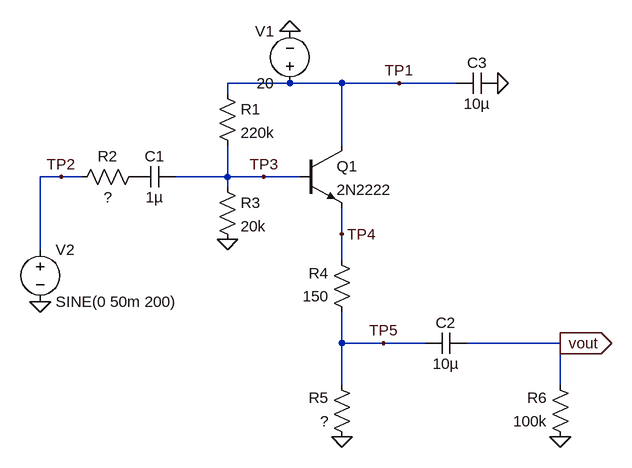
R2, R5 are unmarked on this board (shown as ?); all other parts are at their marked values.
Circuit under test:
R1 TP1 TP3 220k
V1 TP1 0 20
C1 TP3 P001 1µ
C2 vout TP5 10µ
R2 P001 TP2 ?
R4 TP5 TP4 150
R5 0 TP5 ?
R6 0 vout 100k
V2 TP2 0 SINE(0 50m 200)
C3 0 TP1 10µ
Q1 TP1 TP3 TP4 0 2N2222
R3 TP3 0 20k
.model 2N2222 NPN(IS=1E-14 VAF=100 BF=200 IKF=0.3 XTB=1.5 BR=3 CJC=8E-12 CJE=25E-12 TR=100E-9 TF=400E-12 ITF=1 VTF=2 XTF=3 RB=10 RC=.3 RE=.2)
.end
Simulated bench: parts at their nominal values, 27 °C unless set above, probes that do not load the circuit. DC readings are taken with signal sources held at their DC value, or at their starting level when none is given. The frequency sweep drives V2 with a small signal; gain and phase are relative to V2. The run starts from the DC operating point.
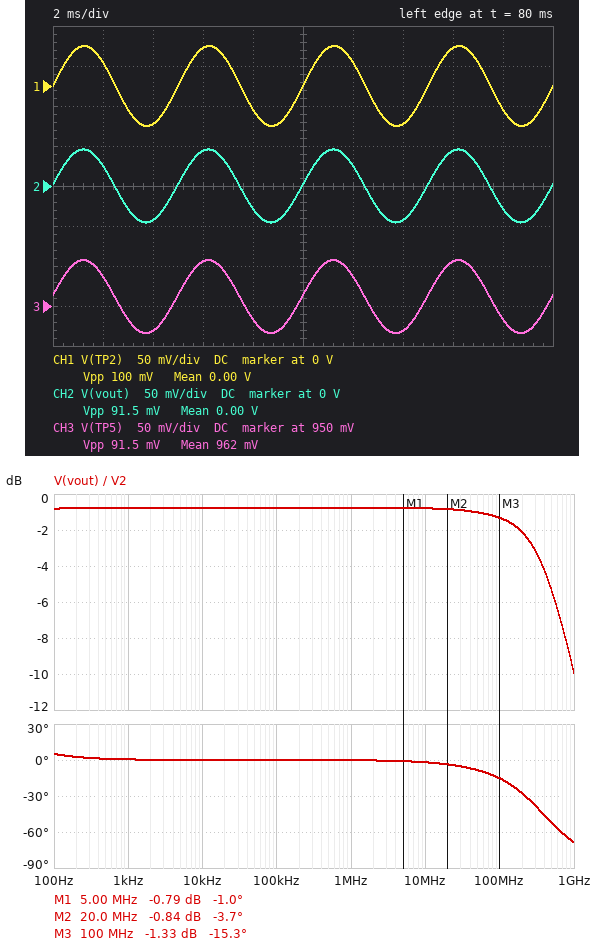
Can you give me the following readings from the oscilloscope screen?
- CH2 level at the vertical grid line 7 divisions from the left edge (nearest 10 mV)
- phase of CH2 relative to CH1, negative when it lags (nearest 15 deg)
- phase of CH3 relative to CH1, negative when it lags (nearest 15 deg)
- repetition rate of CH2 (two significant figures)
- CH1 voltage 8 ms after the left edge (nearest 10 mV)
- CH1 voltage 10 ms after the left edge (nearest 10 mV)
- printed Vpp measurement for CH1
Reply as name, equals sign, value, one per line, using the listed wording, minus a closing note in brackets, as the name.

CH2 level at the vertical grid line 7 divisions from the left edge = -40 mV
phase of CH2 relative to CH1, negative when it lags = 0 deg
phase of CH3 relative to CH1, negative when it lags = 0 deg
repetition rate of CH2 = 200 Hz
CH1 voltage 8 ms after the left edge = -30 mV
CH1 voltage 10 ms after the left edge = 0 V
printed Vpp measurement for CH1 = 100 mV
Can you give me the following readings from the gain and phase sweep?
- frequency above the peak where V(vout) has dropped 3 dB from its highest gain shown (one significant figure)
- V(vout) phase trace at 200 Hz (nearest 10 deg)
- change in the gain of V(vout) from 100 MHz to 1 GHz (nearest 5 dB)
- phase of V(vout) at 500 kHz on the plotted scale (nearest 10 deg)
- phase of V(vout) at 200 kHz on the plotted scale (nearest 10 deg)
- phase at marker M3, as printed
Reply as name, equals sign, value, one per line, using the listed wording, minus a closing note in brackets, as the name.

frequency above the peak where V(vout) has dropped 3 dB from its highest gain shown = 400 MHz
V(vout) phase trace at 200 Hz = 0 deg
change in the gain of V(vout) from 100 MHz to 1 GHz = -10 dB
phase of V(vout) at 500 kHz on the plotted scale = 0 deg
phase of V(vout) at 200 kHz on the plotted scale = 0 deg
phase at marker M3, as printed = -15.3 deg
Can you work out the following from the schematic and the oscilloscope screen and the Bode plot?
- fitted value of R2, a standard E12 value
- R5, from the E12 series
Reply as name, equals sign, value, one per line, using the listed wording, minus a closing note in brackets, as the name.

fitted value of R2, a standard E12 value = 150 Ω
R5, from the E12 series = 2.7 kΩ
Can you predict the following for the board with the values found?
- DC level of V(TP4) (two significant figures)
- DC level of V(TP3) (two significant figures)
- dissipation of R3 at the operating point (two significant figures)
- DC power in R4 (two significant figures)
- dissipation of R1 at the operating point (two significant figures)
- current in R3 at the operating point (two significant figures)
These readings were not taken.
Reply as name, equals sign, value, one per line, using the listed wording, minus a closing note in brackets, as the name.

DC level of V(TP4) = 1.0 V
DC level of V(TP3) = 1.6 V
dissipation of R3 at the operating point = 130 µW
DC power in R4 = 19 µW
dissipation of R1 at the operating point = 1.5 mW
current in R3 at the operating point = 82 µA
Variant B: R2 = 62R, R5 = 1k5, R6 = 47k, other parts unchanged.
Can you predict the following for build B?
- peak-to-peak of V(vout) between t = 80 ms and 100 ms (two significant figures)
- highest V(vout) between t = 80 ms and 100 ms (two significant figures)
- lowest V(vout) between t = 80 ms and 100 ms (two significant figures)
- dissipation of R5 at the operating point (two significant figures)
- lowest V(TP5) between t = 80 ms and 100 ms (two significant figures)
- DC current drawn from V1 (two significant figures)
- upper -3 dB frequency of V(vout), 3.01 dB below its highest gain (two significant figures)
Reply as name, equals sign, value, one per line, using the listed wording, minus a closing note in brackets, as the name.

peak-to-peak of V(vout) between t = 80 ms and 100 ms = 88 mV
highest V(vout) between t = 80 ms and 100 ms = 44 mV
lowest V(vout) between t = 80 ms and 100 ms = -44 mV
dissipation of R5 at the operating point = 530 µW
lowest V(TP5) between t = 80 ms and 100 ms = 850 mV
DC current drawn from V1 = 680 µA
upper -3 dB frequency of V(vout), 3.01 dB below its highest gain = 810 MHz
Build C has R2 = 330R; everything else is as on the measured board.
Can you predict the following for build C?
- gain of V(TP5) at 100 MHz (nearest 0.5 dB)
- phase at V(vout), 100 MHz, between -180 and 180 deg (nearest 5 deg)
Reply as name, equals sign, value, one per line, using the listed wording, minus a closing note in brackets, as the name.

gain of V(TP5) at 100 MHz = -2.5 dB
phase at V(vout), 100 MHz, between -180 and 180 deg = -30 deg
